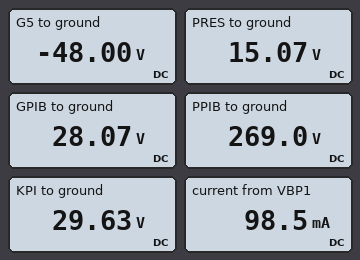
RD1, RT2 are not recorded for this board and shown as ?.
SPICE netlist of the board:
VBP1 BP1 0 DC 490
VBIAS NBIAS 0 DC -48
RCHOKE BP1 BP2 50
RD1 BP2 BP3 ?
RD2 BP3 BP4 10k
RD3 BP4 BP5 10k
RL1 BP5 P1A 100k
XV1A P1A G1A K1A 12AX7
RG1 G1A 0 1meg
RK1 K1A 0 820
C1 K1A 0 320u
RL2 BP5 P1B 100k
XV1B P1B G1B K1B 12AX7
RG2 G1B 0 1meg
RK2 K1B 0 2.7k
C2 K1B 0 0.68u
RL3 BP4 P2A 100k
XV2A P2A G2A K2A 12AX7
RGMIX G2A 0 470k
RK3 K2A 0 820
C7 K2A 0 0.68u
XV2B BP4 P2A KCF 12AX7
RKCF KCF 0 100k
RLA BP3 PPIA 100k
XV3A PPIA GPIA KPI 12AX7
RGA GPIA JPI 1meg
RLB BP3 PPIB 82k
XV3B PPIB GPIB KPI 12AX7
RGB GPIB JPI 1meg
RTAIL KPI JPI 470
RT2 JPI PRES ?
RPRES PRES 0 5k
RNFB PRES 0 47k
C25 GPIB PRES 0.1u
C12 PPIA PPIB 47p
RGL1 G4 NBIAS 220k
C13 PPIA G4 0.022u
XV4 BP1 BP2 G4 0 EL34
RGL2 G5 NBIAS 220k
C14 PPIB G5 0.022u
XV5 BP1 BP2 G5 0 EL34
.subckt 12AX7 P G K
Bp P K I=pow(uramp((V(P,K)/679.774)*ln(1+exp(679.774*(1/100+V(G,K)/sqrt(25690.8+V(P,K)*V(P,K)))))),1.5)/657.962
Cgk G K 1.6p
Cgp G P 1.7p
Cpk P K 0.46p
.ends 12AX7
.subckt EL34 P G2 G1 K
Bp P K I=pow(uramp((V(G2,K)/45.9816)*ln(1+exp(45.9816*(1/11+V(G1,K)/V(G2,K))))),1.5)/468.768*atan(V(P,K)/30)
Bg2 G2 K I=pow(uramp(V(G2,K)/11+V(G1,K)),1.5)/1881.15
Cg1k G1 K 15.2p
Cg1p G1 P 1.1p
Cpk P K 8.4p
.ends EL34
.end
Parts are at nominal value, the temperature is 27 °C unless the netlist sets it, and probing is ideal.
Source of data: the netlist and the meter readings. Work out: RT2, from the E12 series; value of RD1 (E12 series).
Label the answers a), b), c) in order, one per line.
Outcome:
a) 3.9 kΩ
b) 8.2 kΩ
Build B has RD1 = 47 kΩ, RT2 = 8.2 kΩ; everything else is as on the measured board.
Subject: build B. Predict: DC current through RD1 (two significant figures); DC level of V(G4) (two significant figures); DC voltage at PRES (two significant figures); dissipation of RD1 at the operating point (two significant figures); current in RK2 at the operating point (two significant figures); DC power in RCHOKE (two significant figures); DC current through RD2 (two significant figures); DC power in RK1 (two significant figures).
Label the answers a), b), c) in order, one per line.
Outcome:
a) 5.3 mA
b) -48 V
c) 8.6 V
d) 1.3 W
e) 520 µA
f) 1.4 mW
g) 3.4 mA
h) 590 µW
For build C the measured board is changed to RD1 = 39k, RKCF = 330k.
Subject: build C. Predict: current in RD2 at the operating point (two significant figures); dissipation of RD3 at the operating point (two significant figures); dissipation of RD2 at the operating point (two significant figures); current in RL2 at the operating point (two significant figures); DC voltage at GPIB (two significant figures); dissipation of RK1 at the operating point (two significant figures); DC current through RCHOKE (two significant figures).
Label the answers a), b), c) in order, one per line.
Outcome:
a) 3.1 mA
b) 26 mW
c) 98 mW
d) 600 µA
e) 19 V
f) 850 µW
g) 5.4 mA
